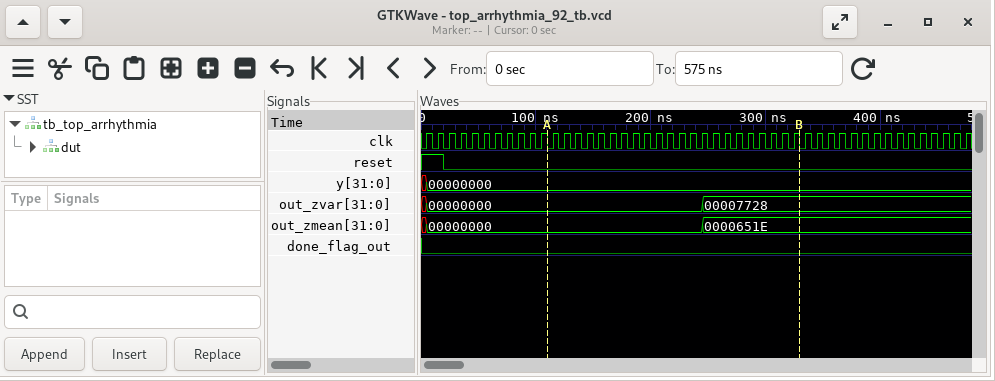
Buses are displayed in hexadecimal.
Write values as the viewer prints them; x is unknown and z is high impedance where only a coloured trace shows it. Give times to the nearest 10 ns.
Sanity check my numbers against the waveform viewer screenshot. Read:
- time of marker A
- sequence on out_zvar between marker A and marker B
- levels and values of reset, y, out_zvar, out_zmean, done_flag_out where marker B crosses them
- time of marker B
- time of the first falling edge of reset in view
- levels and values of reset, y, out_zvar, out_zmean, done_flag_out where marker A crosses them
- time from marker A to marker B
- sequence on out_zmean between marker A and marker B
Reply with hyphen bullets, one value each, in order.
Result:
- 110 ns
- 00000000, 00007728
- reset=0, y=00000000, out_zvar=00007728, out_zmean=0000651E, done_flag_out=0
- 330 ns
- 20 ns
- reset=0, y=00000000, out_zvar=00000000, out_zmean=00000000, done_flag_out=0
- 220 ns
- 00000000, 0000651E
